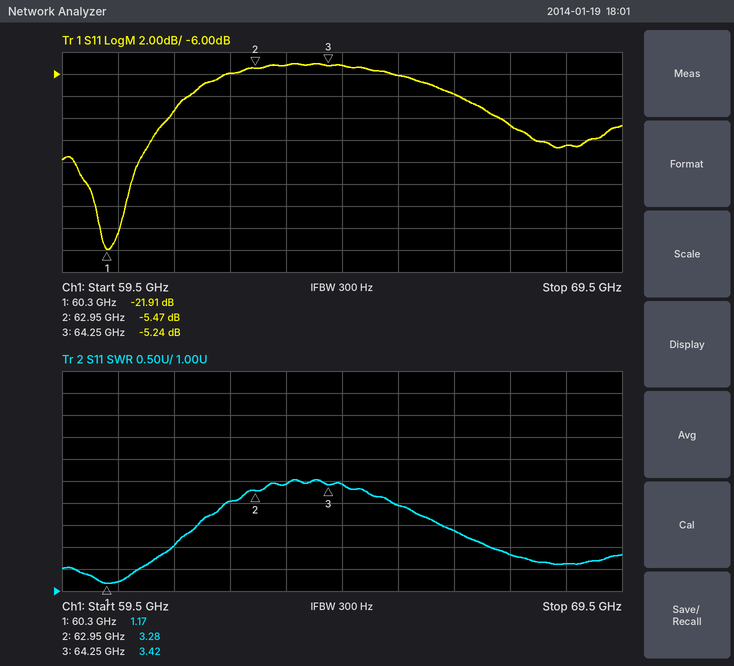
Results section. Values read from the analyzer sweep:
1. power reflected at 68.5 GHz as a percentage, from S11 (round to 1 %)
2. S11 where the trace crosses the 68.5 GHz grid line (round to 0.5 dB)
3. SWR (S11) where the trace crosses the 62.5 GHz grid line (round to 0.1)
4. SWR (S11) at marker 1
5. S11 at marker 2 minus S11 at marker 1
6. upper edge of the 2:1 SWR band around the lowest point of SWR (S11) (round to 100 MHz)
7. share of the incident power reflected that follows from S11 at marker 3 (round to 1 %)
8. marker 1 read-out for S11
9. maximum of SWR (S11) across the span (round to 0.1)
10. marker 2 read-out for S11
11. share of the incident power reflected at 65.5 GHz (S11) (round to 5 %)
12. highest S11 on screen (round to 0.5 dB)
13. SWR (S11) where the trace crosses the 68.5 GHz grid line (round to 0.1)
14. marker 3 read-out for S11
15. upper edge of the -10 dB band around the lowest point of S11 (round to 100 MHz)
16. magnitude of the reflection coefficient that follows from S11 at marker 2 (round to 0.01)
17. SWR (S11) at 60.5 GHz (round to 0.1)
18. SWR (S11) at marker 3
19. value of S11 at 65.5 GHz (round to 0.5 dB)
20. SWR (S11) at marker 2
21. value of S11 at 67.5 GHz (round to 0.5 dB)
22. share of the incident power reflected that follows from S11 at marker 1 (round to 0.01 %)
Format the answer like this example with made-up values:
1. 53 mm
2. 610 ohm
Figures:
1. 6 %
2. -12.5 dB
3. 3.0
4. 1.17
5. 16.44 dB
6. 61.5 GHz
7. 30 %
8. -21.91 dB
9. 3.5
10. -5.47 dB
11. 25 %
12. -5.0 dB
13. 1.6
14. -5.24 dB
15. 61.4 GHz
16. 0.53
17. 1.2
18. 3.42
19. -6.0 dB
20. 3.28
21. -10.5 dB
22. 0.64 %
